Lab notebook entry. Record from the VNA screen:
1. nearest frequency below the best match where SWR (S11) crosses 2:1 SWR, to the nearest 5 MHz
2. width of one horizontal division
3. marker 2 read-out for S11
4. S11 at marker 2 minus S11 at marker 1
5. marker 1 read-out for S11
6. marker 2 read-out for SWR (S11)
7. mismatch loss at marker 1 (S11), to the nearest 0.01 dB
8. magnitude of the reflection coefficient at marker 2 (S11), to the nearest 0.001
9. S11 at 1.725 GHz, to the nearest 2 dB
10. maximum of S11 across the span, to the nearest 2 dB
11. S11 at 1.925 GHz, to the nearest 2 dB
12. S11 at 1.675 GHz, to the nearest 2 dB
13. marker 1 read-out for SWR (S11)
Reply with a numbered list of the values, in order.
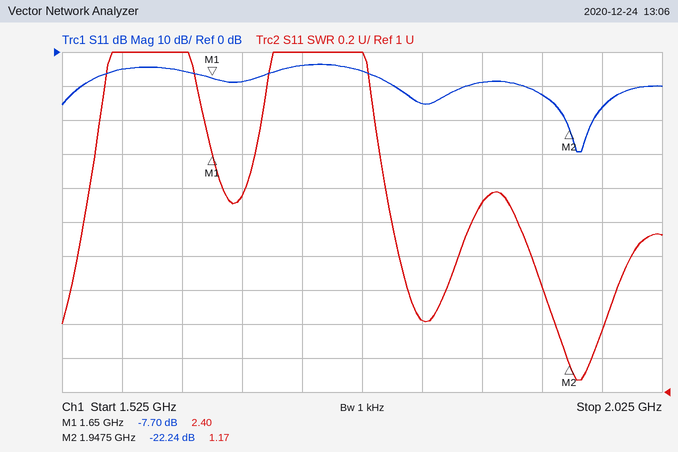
1. 1.905 GHz
2. 50 MHz
3. -22.24 dB
4. -14.54 dB
5. -7.70 dB
6. 1.17
7. 0.81 dB
8. 0.077
9. -4 dB
10. -4 dB
11. -12 dB
12. -8 dB
13. 2.40
